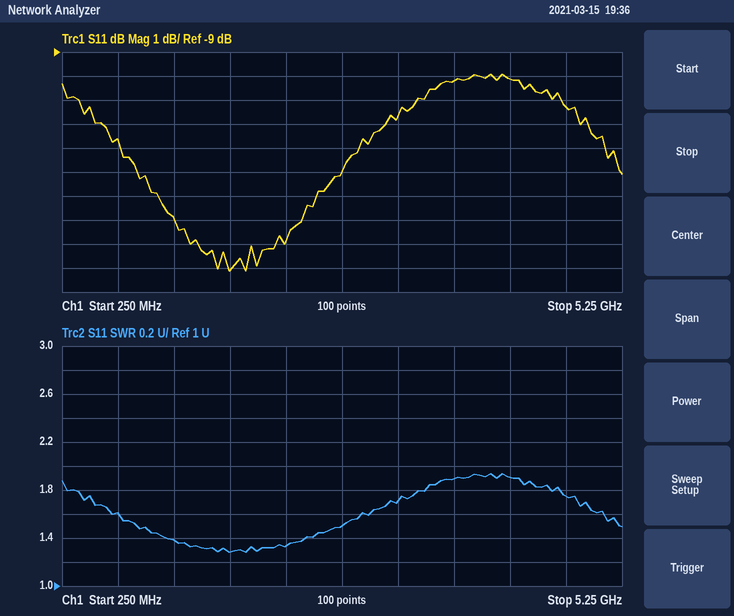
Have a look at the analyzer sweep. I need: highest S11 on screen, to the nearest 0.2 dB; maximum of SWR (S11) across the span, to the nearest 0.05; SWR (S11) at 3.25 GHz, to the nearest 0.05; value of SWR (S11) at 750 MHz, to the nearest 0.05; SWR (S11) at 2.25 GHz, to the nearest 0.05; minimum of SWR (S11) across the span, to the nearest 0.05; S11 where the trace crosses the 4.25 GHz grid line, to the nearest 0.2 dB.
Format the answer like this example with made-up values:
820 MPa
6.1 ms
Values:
-10.0 dB
1.95
1.70
1.60
1.35
1.30
-10.2 dB
